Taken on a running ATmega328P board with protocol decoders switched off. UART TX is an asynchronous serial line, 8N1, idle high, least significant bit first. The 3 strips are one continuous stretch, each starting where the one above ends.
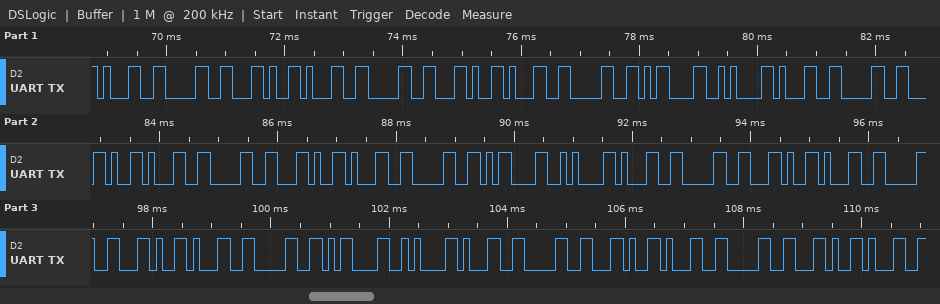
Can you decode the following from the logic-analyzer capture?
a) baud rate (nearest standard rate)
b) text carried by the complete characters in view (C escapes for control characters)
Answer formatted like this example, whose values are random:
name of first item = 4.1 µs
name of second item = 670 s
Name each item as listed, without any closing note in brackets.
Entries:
baud rate = 9600 baud
text carried by the complete characters in view = "10,10,10\r\n10,10,10\r\n10,10,10\r\n10,10,1"
